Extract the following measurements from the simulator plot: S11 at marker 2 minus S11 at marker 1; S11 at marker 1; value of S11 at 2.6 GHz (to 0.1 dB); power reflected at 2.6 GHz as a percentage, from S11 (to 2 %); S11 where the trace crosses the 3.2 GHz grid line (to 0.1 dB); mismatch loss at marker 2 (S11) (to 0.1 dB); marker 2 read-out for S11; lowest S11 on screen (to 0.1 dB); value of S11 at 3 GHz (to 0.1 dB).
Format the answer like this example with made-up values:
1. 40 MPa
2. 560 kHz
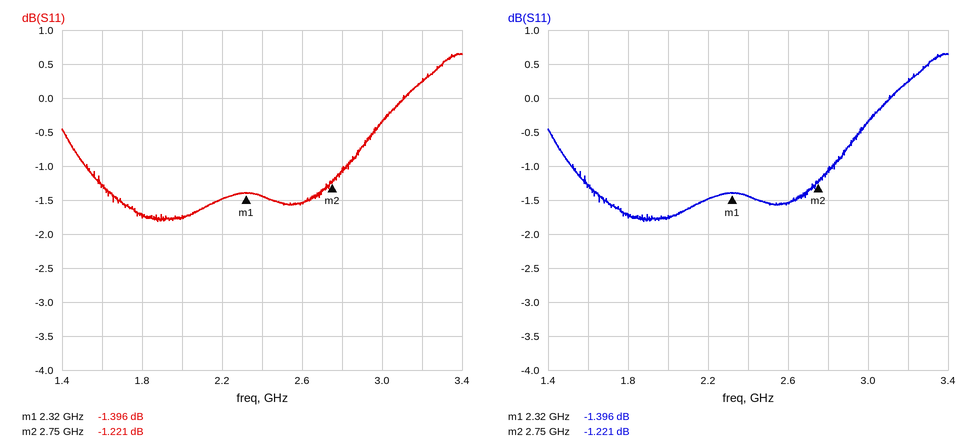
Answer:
1. 0.175 dB
2. -1.396 dB
3. -1.5 dB
4. 70 %
5. 0.2 dB
6. 6.1 dB
7. -1.221 dB
8. -1.8 dB
9. -0.3 dB
